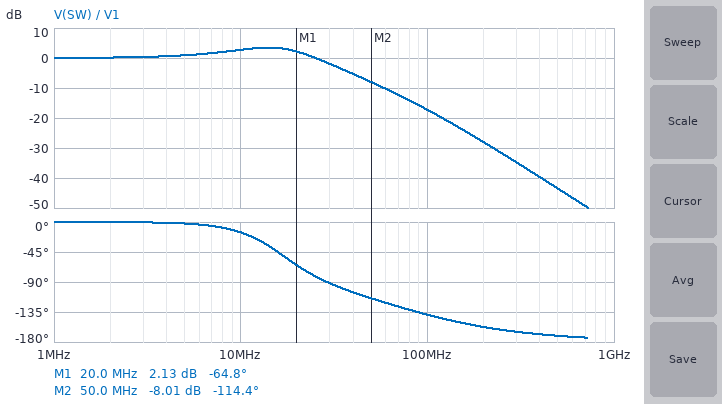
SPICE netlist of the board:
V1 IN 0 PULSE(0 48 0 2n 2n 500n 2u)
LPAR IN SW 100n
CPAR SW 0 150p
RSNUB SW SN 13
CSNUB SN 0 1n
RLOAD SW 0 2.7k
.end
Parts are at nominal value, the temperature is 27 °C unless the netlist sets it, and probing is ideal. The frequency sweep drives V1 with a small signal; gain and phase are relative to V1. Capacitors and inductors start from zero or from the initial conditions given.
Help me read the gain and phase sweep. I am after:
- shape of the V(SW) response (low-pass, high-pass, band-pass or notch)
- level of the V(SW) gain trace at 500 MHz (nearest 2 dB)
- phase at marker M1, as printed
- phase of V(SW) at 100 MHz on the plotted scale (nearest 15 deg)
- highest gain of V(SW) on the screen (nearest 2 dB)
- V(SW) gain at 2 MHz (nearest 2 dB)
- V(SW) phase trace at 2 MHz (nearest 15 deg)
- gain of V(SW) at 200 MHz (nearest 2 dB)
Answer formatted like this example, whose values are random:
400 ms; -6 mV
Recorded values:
low-pass; -44 dB; -64.8 deg; -135 deg; 4 dB; 0 dB; 0 deg; -28 dB
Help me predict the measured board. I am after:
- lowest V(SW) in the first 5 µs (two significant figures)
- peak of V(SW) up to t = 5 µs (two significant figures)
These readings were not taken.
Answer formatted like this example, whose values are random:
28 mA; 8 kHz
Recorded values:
-16 V; 64 V
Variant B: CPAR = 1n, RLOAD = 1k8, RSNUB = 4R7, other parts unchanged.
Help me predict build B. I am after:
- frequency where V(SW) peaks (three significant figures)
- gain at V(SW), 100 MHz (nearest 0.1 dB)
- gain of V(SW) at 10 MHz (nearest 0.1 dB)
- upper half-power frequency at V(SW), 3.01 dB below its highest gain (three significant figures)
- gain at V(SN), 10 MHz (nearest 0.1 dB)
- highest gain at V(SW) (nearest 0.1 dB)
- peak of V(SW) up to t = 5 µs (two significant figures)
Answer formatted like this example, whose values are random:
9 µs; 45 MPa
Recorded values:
11.3 MHz; -32.9 dB; 11.5 dB; 12.3 MHz; 11.1 dB; 15.9 dB; 86 V
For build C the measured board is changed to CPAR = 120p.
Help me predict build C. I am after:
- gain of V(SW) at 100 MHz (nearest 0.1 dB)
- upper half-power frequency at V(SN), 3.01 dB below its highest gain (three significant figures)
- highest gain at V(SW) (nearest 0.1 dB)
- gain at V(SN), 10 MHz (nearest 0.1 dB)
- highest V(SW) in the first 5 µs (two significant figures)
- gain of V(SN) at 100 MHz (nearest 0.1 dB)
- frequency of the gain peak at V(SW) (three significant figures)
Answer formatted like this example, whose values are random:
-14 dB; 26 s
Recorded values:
-16.2 dB; 18.3 MHz; 3.2 dB; 0.4 dB; 63 V; -34.5 dB; 13.9 MHz
